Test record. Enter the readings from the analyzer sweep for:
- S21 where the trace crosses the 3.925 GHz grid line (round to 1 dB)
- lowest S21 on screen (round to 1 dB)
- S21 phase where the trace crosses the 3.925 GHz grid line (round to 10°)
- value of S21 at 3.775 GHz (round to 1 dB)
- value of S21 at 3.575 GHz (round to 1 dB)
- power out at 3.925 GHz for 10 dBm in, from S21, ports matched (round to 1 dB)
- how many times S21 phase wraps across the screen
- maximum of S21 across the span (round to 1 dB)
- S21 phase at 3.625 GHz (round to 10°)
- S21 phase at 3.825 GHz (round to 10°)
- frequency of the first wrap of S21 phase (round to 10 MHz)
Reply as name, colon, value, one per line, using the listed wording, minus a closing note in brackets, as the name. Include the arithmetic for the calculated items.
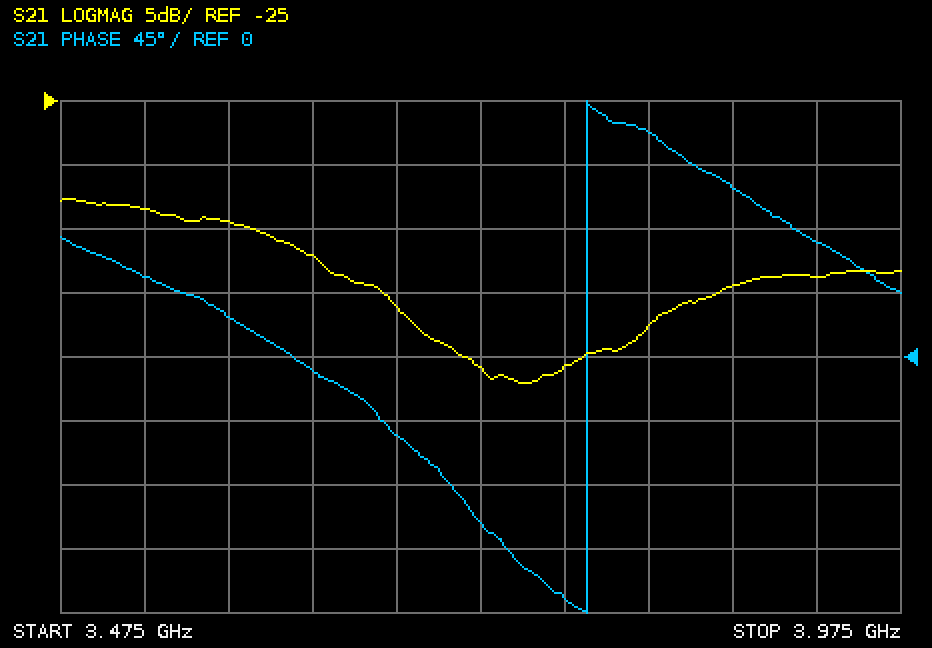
S21 where the trace crosses the 3.925 GHz grid line: -39 dB
lowest S21 on screen: -47 dB
S21 phase where the trace crosses the 3.925 GHz grid line: 80°
value of S21 at 3.775 GHz: -46 dB
value of S21 at 3.575 GHz: -34 dB
power out at 3.925 GHz for 10 dBm in, from S21, ports matched: 10 dBm + (-39 dB) = -29 dBm
how many times S21 phase wraps across the screen: 1
maximum of S21 across the span: -33 dB
S21 phase at 3.625 GHz: -10°
S21 phase at 3.825 GHz: 160°
frequency of the first wrap of S21 phase: 3.79 GHz
